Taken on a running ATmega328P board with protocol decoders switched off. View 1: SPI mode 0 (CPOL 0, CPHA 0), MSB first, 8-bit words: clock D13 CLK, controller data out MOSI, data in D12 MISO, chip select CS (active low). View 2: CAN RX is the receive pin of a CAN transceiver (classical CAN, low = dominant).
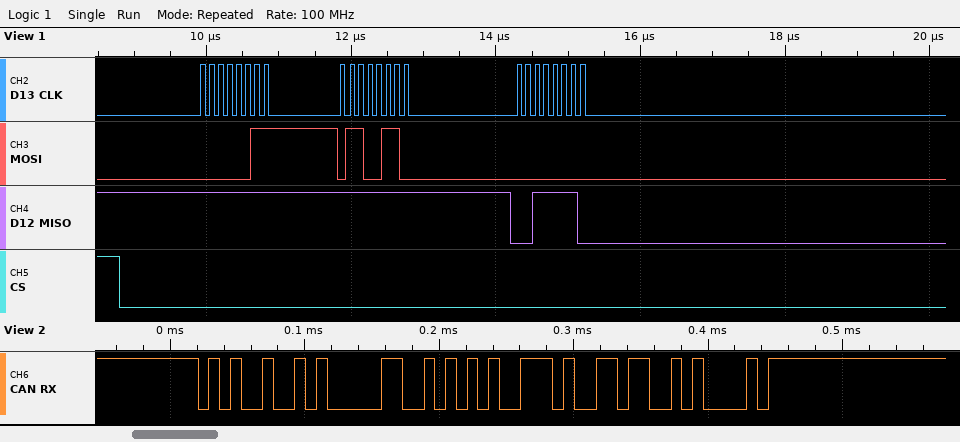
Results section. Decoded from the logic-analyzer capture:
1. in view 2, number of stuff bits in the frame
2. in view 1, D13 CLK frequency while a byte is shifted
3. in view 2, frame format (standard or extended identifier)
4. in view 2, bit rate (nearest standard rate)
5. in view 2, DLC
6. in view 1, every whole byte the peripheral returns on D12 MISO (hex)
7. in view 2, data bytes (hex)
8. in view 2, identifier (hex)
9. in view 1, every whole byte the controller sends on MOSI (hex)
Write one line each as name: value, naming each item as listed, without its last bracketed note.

in view 2, number of stuff bits in the frame: 1
in view 1, D13 CLK frequency while a byte is shifted: 8 MHz
in view 2, frame format: standard
in view 2, bit rate: 125 kbit/s
in view 2, DLC: 2
in view 1, every whole byte the peripheral returns on D12 MISO: FF FF 3E
in view 2, data bytes: 55 3A
in view 2, identifier: 0x525
in view 1, every whole byte the controller sends on MOSI: 03 66 00
